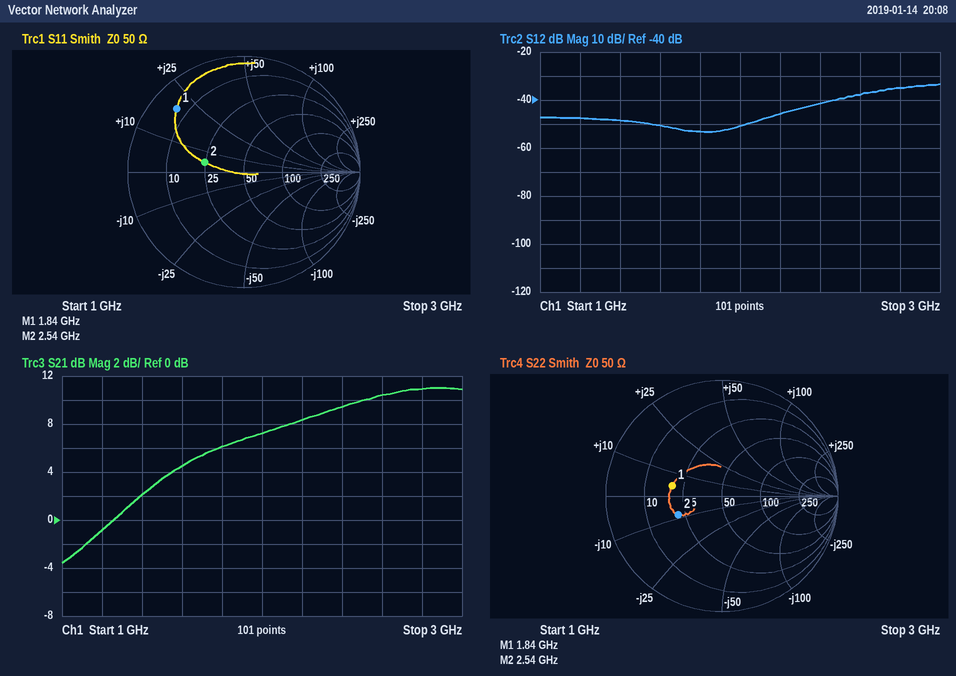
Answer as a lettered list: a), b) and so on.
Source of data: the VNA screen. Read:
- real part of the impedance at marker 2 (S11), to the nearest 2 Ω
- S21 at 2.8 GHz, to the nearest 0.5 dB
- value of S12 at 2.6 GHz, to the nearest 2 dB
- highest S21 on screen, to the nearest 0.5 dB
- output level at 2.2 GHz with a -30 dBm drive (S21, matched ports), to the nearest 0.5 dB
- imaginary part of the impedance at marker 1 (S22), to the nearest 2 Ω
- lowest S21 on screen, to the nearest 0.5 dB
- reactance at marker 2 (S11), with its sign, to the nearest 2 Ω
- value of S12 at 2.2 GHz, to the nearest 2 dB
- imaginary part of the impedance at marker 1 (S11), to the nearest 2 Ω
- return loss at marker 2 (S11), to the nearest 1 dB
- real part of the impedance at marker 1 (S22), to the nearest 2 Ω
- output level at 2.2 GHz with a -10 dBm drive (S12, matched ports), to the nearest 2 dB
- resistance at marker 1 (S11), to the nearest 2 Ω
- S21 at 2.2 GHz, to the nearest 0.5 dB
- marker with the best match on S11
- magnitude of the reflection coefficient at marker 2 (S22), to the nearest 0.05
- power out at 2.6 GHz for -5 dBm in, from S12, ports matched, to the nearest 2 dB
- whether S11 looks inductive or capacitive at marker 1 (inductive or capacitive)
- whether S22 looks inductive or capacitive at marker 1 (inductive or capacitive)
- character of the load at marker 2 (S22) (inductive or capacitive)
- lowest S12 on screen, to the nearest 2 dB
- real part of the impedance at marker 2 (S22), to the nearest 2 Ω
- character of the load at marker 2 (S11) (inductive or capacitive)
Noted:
a) 24 Ω
b) 11.0 dB
c) -38 dB
d) 11.0 dB
e) -21.5 dBm
f) +4 Ω
g) -3.5 dB
h) +4 Ω
i) -46 dB
j) +20 Ω
k) 9 dB
l) 20 Ω
m) -56 dBm
n) 6 Ω
o) 8.5 dB
p) marker 2
q) 0.40
r) -42 dBm
s) inductive
t) inductive
u) capacitive
v) -54 dB
w) 22 Ω
x) inductive
